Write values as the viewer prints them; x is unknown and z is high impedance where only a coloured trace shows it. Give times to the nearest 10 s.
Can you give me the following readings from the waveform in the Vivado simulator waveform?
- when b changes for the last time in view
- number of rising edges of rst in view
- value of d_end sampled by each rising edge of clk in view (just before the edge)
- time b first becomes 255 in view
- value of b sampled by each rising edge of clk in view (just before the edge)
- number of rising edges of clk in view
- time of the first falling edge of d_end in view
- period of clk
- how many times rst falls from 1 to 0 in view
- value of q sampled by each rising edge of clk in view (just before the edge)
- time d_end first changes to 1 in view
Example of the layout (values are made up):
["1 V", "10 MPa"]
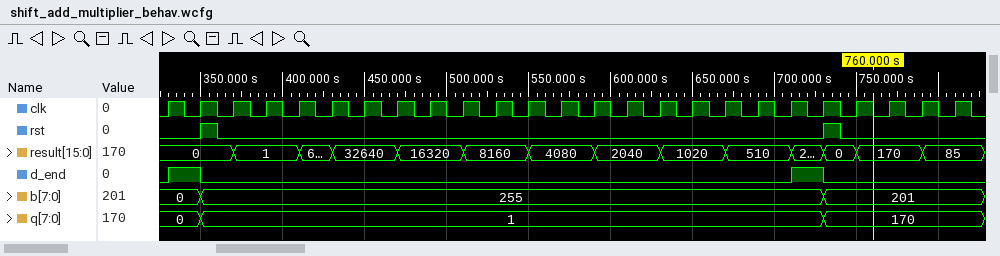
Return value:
["730 s", "2", "0 1 0 0 0 0 0 0 0 0 0 0 0 0 0 0 0 0 0 0 1 0 0 0 0", "350 s", "0, 0, 255, 255, 255, 255, 255, 255, 255, 255, 255, 255, 255, 255, 255, 255, 255, 255, 255, 255, 255, 201, 201, 201, 201", "25", "350 s", "20 s", "2", "0, 0, 1, 1, 1, 1, 1, 1, 1, 1, 1, 1, 1, 1, 1, 1, 1, 1, 1, 1, 1, 170, 170, 170, 170", "330 s"]
